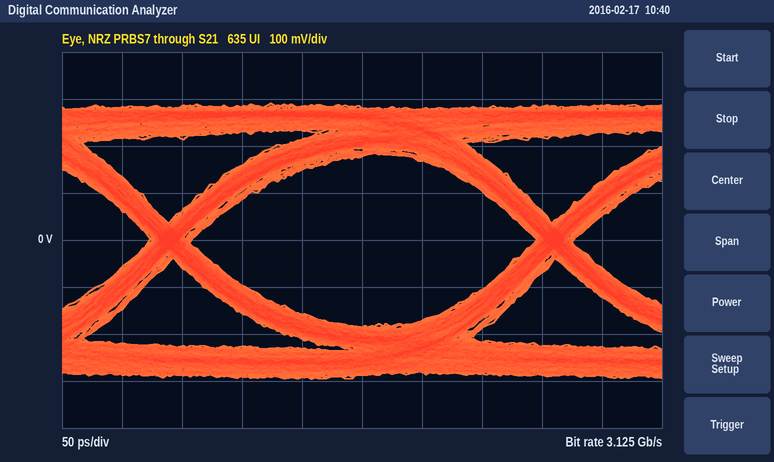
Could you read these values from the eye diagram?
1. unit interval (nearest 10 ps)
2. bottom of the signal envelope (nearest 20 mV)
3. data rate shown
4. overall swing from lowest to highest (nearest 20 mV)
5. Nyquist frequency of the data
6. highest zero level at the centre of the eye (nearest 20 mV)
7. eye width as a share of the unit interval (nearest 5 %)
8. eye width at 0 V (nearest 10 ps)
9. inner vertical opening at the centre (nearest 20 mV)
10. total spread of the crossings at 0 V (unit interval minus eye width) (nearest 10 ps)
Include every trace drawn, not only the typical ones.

320 ps
-300 mV
3.125 Gb/s
580 mV
1.5625 GHz
-180 mV
90 %
290 ps
360 mV
30 ps
